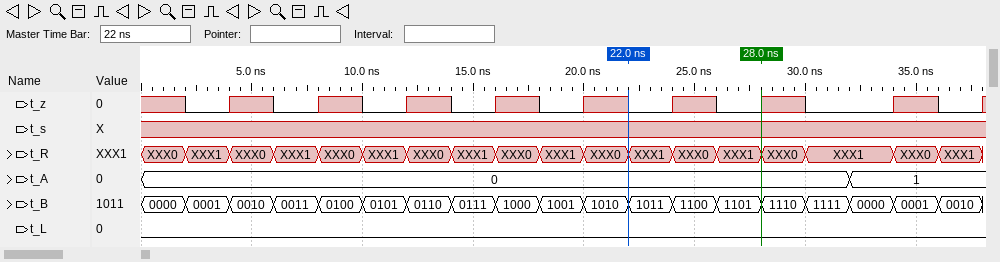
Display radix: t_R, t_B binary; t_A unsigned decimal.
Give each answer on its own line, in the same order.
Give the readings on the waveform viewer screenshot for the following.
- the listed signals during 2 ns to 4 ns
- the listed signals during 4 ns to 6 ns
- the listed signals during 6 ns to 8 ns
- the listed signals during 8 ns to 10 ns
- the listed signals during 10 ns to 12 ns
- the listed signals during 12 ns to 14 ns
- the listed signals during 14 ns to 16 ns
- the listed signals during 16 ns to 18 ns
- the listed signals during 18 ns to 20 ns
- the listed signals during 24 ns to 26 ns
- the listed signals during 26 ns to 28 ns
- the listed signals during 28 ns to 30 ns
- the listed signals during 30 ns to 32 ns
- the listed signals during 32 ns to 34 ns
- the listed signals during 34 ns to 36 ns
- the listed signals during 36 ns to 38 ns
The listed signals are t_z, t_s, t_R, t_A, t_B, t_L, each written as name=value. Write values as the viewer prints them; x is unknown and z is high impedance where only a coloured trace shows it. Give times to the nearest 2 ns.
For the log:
t_z=0, t_s=x, t_R=XXX1, t_A=0, t_B=0001, t_L=0
t_z=x, t_s=x, t_R=XXX0, t_A=0, t_B=0010, t_L=0
t_z=0, t_s=x, t_R=XXX1, t_A=0, t_B=0011, t_L=0
t_z=x, t_s=x, t_R=XXX0, t_A=0, t_B=0100, t_L=0
t_z=0, t_s=x, t_R=XXX1, t_A=0, t_B=0101, t_L=0
t_z=x, t_s=x, t_R=XXX0, t_A=0, t_B=0110, t_L=0
t_z=0, t_s=x, t_R=XXX1, t_A=0, t_B=0111, t_L=0
t_z=x, t_s=x, t_R=XXX0, t_A=0, t_B=1000, t_L=0
t_z=0, t_s=x, t_R=XXX1, t_A=0, t_B=1001, t_L=0
t_z=x, t_s=x, t_R=XXX0, t_A=0, t_B=1100, t_L=0
t_z=0, t_s=x, t_R=XXX1, t_A=0, t_B=1101, t_L=0
t_z=x, t_s=x, t_R=XXX0, t_A=0, t_B=1110, t_L=0
t_z=0, t_s=x, t_R=XXX1, t_A=0, t_B=1111, t_L=0
t_z=0, t_s=x, t_R=XXX1, t_A=1, t_B=0000, t_L=0
t_z=x, t_s=x, t_R=XXX0, t_A=1, t_B=0001, t_L=0
t_z=0, t_s=x, t_R=XXX1, t_A=1, t_B=0010, t_L=0
